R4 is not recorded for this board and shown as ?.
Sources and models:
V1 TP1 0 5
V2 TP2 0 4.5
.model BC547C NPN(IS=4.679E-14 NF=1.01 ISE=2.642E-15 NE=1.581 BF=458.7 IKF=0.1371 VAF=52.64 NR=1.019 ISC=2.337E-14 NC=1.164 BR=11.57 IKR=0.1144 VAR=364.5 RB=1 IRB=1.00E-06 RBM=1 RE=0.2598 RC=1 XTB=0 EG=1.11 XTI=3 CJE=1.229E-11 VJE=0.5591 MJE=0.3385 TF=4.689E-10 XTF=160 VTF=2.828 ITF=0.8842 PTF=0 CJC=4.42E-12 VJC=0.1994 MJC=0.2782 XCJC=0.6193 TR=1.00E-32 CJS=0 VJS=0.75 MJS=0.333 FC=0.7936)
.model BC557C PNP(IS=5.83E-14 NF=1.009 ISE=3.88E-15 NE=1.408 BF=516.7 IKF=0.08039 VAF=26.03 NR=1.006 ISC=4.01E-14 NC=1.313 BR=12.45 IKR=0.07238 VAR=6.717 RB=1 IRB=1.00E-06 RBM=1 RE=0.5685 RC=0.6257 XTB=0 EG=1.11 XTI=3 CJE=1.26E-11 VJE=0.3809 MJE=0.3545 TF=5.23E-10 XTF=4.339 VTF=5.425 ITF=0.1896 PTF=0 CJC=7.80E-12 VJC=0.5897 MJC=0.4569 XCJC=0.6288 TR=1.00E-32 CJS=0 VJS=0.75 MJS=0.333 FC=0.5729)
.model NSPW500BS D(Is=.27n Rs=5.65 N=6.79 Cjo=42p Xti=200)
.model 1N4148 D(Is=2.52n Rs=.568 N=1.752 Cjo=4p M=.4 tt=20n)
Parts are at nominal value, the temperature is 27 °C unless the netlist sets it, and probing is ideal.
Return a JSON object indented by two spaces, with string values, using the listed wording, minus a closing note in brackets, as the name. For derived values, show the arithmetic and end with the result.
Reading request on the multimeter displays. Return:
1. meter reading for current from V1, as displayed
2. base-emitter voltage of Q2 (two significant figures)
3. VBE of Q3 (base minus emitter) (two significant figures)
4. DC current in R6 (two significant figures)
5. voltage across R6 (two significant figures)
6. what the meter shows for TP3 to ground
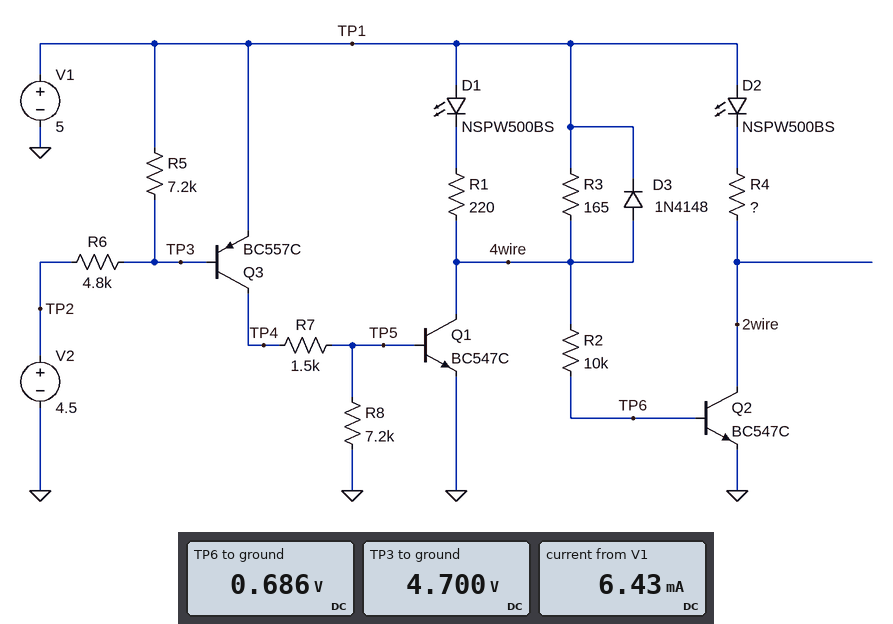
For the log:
{
  "meter reading for current from V1, as displayed": "6.43 mA",
  "base-emitter voltage of Q2": "686 mV = 690 mV",
  "VBE of Q3 (base minus emitter)": "4.7 V - 5 V = -300 mV",
  "DC current in R6": "(4.7 V - 4.5 V) / 4.8 kΩ = 42 µA",
  "voltage across R6": "4.7 V - 4.5 V = 200 mV",
  "what the meter shows for TP3 to ground": "4.700 V"
}
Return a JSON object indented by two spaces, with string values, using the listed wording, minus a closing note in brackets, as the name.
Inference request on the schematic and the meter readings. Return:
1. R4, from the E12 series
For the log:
{
  "R4, from the E12 series": "330 Ω"
}
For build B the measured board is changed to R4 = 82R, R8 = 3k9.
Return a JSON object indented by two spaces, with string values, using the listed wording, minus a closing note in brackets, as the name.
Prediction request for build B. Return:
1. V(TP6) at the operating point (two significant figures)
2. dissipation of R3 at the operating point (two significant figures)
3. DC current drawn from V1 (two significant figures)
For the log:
{
  "V(TP6) at the operating point": "710 mV",
  "dissipation of R3 at the operating point": "29 µW",
  "DC current drawn from V1": "20 mA"
}
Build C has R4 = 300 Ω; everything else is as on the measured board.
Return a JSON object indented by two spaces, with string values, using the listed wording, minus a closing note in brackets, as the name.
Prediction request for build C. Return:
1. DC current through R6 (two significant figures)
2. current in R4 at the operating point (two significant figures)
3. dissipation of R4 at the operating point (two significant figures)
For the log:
{
  "DC current through R6": "42 µA",
  "current in R4 at the operating point": "6.5 mA",
  "dissipation of R4 at the operating point": "13 mW"
}
